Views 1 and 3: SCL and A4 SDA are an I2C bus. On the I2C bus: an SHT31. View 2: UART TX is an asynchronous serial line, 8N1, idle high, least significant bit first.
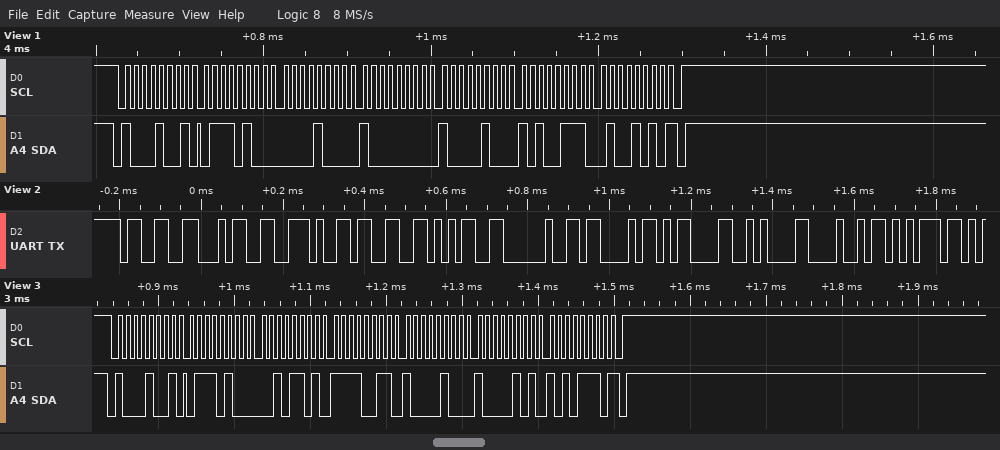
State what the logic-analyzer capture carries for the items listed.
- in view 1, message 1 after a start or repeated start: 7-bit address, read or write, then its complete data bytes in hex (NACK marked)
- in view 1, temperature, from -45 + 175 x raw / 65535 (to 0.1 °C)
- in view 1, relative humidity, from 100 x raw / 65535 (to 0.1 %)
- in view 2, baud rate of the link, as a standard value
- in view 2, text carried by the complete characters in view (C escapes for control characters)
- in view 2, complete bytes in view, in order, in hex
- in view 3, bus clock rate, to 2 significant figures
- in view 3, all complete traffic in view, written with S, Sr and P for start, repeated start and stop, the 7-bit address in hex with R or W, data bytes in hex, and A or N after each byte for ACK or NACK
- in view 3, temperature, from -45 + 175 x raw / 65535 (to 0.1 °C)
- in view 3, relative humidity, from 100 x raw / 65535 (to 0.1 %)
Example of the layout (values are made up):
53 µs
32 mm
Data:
0x44 read: 74 08 80 84 A7 4A NACK
34.3 °C
51.8 %
57600 baud
"34.35 C\r\nHu"
33 34 2E 33 35 20 43 0D 0A 48 75
100 kHz
S 44R A 74 A 2D A F3 A 84 A 85 A AE N P
34.4 °C
51.8 %
